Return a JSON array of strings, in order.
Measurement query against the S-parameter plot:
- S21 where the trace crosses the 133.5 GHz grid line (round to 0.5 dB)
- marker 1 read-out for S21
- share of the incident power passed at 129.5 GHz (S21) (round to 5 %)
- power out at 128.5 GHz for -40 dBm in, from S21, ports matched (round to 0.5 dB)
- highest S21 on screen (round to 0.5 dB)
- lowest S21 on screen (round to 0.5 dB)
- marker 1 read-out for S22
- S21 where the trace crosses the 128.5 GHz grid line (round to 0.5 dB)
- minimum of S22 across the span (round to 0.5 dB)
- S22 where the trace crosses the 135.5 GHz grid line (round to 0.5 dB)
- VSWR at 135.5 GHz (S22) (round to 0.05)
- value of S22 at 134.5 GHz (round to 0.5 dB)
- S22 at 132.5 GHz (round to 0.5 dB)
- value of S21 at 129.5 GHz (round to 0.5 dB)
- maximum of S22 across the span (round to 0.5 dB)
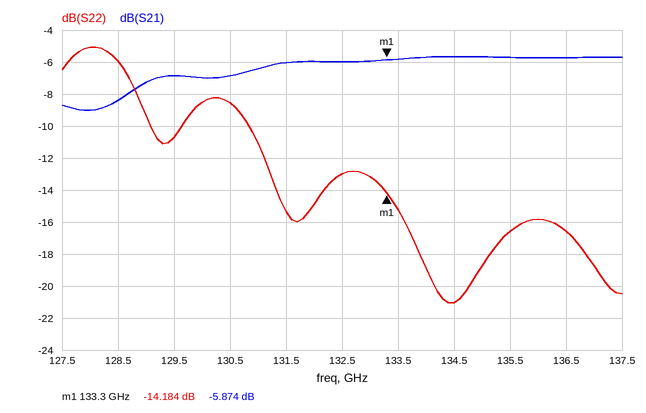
["-6.0 dB", "-5.874 dB", "20 %", "-48.5 dBm", "-5.5 dB", "-9.0 dB", "-14.184 dB", "-8.5 dB", "-21.0 dB", "-16.5 dB", "1.35", "-21.0 dB", "-13.0 dB", "-7.0 dB", "-5.0 dB"]
